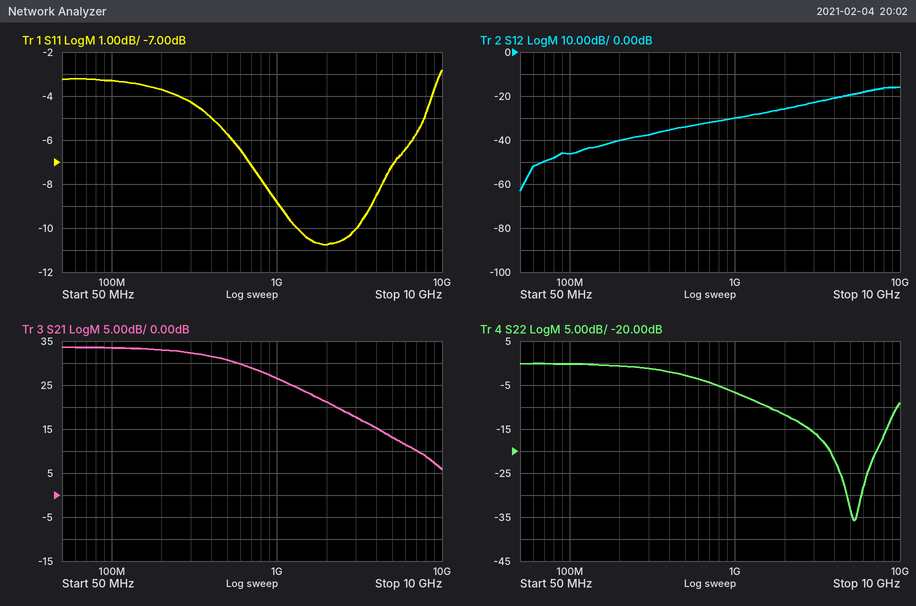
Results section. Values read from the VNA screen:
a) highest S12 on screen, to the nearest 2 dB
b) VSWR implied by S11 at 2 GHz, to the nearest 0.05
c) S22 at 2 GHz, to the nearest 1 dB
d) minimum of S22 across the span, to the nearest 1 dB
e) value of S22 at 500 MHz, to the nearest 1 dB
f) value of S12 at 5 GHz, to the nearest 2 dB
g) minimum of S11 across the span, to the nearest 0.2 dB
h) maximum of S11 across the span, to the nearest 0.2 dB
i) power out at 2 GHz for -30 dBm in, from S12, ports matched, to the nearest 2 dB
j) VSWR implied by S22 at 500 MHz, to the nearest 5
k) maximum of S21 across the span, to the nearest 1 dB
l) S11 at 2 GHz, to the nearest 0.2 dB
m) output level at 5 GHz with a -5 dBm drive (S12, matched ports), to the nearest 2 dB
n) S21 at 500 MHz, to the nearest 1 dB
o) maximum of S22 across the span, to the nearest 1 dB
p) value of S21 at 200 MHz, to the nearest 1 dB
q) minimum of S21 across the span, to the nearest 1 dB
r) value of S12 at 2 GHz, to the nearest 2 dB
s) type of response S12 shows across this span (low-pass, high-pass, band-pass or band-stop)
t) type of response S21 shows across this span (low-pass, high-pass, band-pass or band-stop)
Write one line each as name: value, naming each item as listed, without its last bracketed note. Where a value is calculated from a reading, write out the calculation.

highest S12 on screen, to the nearest 2 dB: -16 dB
VSWR implied by S11 at 2 GHz, to the nearest 0.05: |Γ| = 10^(-10.8/20) = 0.2884; VSWR = (1 + 0.2884)/(1 − 0.2884) ≈ 1.81, so 1.80 to the nearest 0.05
S22 at 2 GHz, to the nearest 1 dB: -12 dB
minimum of S22 across the span, to the nearest 1 dB: -36 dB
value of S22 at 500 MHz, to the nearest 1 dB: -3 dB
value of S12 at 5 GHz, to the nearest 2 dB: -20 dB
minimum of S11 across the span, to the nearest 0.2 dB: -10.8 dB
maximum of S11 across the span, to the nearest 0.2 dB: -2.8 dB
power out at 2 GHz for -30 dBm in, from S12, ports matched, to the nearest 2 dB: -30 dBm + (-26 dB) = -56 dBm
VSWR implied by S22 at 500 MHz, to the nearest 5: |Γ| = 10^(-3/20) = 0.7079; VSWR = (1 + 0.7079)/(1 − 0.7079) ≈ 5.85, so 5 to the nearest 5
maximum of S21 across the span, to the nearest 1 dB: 34 dB
S11 at 2 GHz, to the nearest 0.2 dB: -10.8 dB
output level at 5 GHz with a -5 dBm drive (S12, matched ports), to the nearest 2 dB: -5 dBm + (-20 dB) = -24 dBm
S21 at 500 MHz, to the nearest 1 dB: 31 dB
maximum of S22 across the span, to the nearest 1 dB: 0 dB
value of S21 at 200 MHz, to the nearest 1 dB: 33 dB
minimum of S21 across the span, to the nearest 1 dB: 6 dB
value of S12 at 2 GHz, to the nearest 2 dB: -26 dB
type of response S12 shows across this span: high-pass
type of response S21 shows across this span: low-pass
